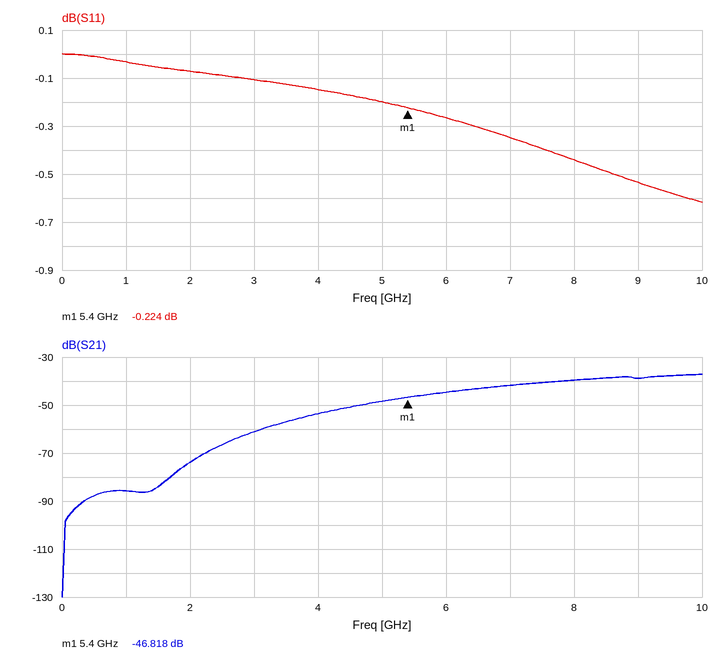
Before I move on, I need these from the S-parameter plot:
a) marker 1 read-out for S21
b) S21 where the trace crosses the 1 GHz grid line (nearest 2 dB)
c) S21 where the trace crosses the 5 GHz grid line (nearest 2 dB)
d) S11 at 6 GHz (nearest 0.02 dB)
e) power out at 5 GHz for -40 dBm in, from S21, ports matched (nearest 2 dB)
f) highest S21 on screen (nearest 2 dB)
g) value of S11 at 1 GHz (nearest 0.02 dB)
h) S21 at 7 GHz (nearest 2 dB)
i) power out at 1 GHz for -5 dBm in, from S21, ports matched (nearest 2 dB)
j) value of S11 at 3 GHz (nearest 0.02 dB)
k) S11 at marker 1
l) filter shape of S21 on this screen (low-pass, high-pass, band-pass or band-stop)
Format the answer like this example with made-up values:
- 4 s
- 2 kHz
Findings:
- -46.818 dB
- -86 dB
- -48 dB
- -0.26 dB
- -88 dBm
- -38 dB
- -0.04 dB
- -42 dB
- -90 dBm
- -0.10 dB
- -0.224 dB
- high-pass
